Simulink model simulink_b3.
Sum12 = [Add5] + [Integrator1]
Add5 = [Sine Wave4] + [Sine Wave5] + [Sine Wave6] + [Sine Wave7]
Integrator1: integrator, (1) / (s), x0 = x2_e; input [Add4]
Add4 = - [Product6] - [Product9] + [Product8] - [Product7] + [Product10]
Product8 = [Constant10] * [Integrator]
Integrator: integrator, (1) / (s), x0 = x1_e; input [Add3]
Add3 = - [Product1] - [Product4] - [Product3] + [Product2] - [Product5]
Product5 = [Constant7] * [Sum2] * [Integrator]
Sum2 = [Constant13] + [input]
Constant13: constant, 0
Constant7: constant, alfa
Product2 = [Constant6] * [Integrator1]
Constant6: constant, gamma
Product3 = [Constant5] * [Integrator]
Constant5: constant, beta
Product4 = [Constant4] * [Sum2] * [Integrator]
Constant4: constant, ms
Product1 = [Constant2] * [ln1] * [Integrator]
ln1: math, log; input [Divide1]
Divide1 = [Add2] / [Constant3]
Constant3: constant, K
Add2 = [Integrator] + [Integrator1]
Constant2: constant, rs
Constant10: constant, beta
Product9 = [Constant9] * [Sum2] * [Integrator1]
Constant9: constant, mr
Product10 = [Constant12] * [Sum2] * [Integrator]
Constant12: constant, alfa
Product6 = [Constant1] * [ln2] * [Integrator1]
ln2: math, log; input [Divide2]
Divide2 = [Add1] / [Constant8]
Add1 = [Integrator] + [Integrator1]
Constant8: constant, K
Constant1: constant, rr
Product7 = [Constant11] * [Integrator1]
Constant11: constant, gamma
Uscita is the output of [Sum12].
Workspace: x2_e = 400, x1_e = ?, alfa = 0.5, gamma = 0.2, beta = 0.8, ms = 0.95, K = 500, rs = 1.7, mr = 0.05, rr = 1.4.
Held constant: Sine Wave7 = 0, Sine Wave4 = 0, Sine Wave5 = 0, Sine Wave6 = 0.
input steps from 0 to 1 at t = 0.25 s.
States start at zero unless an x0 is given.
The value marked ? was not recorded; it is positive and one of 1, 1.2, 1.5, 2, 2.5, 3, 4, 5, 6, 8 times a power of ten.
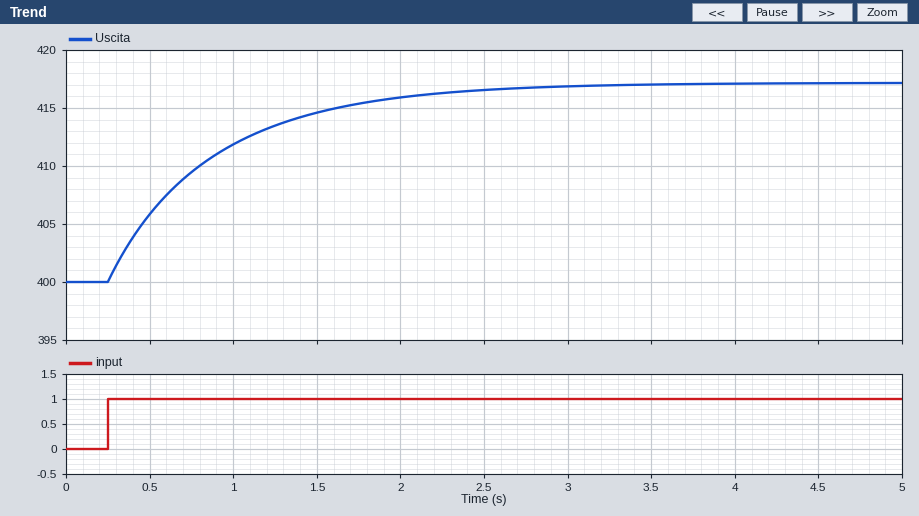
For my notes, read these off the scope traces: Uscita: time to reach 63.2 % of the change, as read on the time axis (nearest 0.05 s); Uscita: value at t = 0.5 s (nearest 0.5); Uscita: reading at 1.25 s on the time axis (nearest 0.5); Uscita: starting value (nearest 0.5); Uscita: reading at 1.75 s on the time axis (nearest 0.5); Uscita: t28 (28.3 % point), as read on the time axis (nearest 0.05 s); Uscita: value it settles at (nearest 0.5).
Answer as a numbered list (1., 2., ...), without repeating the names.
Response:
1. 0.90 s
2. 406.0
3. 413.5
4. 400.0
5. 415.5
6. 0.45 s
7. 417.0
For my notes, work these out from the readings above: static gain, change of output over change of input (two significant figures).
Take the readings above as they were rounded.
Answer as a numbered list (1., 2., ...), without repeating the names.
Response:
1. 17
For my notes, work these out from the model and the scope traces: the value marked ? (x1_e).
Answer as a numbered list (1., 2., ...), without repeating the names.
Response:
1. 100
